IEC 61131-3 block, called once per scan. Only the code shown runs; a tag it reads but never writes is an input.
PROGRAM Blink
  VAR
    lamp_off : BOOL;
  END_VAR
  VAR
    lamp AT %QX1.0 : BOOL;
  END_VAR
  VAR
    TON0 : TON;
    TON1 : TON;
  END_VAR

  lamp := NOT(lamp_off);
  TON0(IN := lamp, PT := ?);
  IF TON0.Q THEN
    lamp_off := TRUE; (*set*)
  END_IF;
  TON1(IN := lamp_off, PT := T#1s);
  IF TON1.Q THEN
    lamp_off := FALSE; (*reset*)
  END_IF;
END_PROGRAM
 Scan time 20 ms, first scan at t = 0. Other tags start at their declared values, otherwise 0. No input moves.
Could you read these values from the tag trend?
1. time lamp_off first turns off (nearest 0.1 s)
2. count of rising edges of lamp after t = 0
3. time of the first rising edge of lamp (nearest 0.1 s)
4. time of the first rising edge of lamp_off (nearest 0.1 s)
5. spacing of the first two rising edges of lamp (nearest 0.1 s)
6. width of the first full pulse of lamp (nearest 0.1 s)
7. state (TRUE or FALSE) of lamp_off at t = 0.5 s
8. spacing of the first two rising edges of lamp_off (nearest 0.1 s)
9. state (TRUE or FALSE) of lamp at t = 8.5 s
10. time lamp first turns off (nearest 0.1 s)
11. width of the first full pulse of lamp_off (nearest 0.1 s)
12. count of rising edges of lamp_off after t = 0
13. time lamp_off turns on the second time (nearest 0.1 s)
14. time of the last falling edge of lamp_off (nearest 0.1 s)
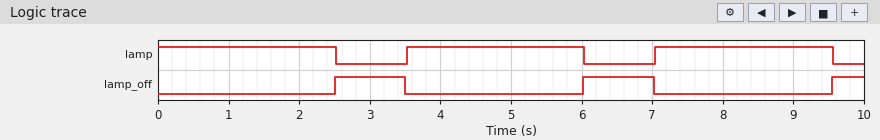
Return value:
3.5 s
2
3.5 s
2.5 s
3.5 s
2.5 s
FALSE
3.5 s
TRUE
2.5 s
1.0 s
3
6.0 s
7.0 s
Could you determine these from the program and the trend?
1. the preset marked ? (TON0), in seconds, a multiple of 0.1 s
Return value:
2.5 s
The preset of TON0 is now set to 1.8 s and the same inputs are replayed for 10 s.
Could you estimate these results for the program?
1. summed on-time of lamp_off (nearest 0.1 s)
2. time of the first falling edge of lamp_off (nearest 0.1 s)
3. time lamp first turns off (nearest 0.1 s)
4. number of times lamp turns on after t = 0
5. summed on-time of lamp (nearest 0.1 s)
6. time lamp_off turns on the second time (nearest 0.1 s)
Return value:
3.0 s
2.8 s
1.8 s
3
7.0 s
4.6 s
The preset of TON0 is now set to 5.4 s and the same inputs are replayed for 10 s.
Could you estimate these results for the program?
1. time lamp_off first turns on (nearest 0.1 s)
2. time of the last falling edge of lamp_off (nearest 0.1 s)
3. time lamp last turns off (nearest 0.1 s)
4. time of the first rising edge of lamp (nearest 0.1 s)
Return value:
5.4 s
6.4 s
5.4 s
6.4 s
